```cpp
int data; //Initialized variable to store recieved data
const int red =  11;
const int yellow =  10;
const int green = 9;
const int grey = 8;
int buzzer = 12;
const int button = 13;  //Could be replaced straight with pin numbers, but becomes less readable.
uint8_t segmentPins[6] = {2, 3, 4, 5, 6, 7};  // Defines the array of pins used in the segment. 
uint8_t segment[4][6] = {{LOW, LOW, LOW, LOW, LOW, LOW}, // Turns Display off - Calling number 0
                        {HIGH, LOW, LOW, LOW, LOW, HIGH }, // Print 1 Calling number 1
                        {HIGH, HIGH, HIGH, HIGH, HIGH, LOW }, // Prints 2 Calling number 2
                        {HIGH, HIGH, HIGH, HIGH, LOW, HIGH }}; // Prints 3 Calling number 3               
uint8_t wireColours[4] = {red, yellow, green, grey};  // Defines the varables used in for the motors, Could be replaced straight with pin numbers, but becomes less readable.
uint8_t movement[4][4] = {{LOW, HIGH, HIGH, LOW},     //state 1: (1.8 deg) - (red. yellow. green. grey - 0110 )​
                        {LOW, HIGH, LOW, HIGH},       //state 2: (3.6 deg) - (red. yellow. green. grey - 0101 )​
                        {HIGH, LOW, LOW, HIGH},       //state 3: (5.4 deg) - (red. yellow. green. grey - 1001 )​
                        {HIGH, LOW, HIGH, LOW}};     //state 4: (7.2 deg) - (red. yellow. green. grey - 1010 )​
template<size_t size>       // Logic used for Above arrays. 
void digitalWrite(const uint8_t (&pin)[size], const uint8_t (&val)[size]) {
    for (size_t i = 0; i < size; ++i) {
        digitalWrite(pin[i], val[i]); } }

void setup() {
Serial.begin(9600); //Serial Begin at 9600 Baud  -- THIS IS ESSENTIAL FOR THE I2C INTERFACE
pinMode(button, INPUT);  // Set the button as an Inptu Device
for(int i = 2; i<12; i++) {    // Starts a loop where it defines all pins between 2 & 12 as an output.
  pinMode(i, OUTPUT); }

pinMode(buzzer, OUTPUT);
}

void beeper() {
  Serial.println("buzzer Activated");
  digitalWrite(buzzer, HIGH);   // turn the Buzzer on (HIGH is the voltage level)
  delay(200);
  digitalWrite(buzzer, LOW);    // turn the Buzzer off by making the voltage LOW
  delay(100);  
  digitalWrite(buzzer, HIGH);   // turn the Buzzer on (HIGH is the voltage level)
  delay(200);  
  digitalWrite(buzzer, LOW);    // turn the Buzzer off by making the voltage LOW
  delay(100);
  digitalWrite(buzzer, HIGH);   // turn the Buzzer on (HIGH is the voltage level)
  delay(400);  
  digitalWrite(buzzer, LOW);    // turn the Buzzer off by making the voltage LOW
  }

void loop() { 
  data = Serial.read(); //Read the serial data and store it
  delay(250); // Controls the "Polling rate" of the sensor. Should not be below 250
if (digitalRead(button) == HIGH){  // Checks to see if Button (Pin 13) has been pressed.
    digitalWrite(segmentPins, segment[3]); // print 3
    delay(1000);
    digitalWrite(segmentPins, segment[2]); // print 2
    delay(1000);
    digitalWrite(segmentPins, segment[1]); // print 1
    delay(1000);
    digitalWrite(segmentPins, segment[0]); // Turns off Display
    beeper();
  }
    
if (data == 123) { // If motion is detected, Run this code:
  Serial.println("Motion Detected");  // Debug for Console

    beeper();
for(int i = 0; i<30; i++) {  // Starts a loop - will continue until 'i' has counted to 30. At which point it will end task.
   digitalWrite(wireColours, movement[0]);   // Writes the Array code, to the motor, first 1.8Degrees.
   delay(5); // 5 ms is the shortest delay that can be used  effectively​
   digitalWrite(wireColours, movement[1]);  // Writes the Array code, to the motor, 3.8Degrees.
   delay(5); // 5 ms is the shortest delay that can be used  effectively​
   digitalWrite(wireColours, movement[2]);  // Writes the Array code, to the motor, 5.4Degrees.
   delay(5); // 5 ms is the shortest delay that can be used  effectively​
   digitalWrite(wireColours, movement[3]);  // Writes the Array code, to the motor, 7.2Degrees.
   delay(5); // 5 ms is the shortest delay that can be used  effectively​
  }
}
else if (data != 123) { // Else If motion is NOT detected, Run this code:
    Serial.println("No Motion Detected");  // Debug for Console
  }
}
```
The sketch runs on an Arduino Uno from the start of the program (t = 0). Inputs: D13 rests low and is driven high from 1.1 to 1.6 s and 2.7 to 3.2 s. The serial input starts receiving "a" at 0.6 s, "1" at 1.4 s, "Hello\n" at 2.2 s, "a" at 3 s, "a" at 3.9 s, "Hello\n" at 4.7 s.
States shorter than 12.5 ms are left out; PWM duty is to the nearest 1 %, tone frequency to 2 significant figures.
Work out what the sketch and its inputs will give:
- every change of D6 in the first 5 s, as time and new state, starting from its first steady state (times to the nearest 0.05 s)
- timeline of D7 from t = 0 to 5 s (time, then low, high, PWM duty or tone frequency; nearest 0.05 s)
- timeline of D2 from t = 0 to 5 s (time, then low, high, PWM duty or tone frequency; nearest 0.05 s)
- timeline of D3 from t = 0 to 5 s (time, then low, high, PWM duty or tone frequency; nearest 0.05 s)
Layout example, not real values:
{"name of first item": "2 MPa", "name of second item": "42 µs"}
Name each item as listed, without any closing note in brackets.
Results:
{"every change of D6 in the first 5 s, as time and new state, starting from its first steady state": "0 s low; 2.25 s high; 3.25 s low", "timeline of D7 from t = 0 to 5 s": "0 s low; 1.25 s high; 2.25 s low; 3.25 s high; 4.25 s low", "timeline of D2 from t = 0 to 5 s": "0 s low; 1.25 s high; 4.25 s low", "timeline of D3 from t = 0 to 5 s": "0 s low; 1.25 s high; 3.25 s low"}
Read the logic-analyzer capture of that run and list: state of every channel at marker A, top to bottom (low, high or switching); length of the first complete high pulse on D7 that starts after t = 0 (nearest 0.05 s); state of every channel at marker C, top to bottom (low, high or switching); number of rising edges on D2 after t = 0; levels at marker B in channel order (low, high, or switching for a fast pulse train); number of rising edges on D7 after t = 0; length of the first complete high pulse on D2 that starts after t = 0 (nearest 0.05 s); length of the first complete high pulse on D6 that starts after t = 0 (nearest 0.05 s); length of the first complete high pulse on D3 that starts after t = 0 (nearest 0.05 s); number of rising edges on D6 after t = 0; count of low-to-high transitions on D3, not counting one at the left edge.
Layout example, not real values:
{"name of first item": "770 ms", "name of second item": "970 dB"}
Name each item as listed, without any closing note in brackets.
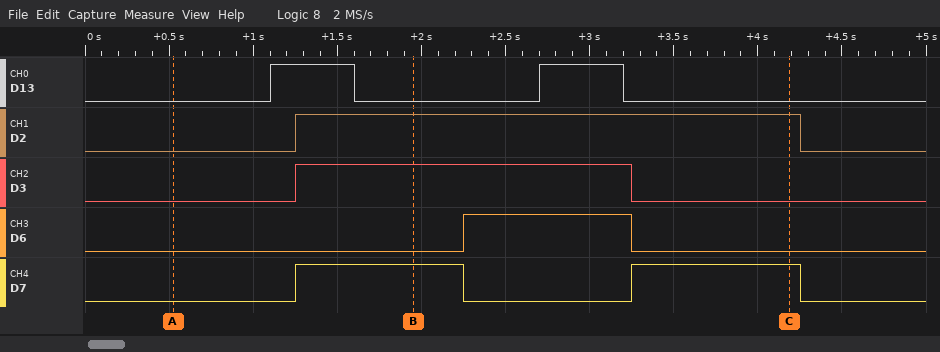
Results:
{"state of every channel at marker A, top to bottom": "D13 low, D2 low, D3 low, D6 low, D7 low", "length of the first complete high pulse on D7 that starts after t = 0": "1.00 s", "state of every channel at marker C, top to bottom": "D13 low, D2 high, D3 low, D6 low, D7 high", "number of rising edges on D2 after t = 0": "1", "levels at marker B in channel order": "D13 low, D2 high, D3 high, D6 low, D7 high", "number of rising edges on D7 after t = 0": "2", "length of the first complete high pulse on D2 that starts after t = 0": "3.00 s", "length of the first complete high pulse on D6 that starts after t = 0": "1.00 s", "length of the first complete high pulse on D3 that starts after t = 0": "2.00 s", "number of rising edges on D6 after t = 0": "1", "count of low-to-high transitions on D3, not counting one at the left edge": "1"}
